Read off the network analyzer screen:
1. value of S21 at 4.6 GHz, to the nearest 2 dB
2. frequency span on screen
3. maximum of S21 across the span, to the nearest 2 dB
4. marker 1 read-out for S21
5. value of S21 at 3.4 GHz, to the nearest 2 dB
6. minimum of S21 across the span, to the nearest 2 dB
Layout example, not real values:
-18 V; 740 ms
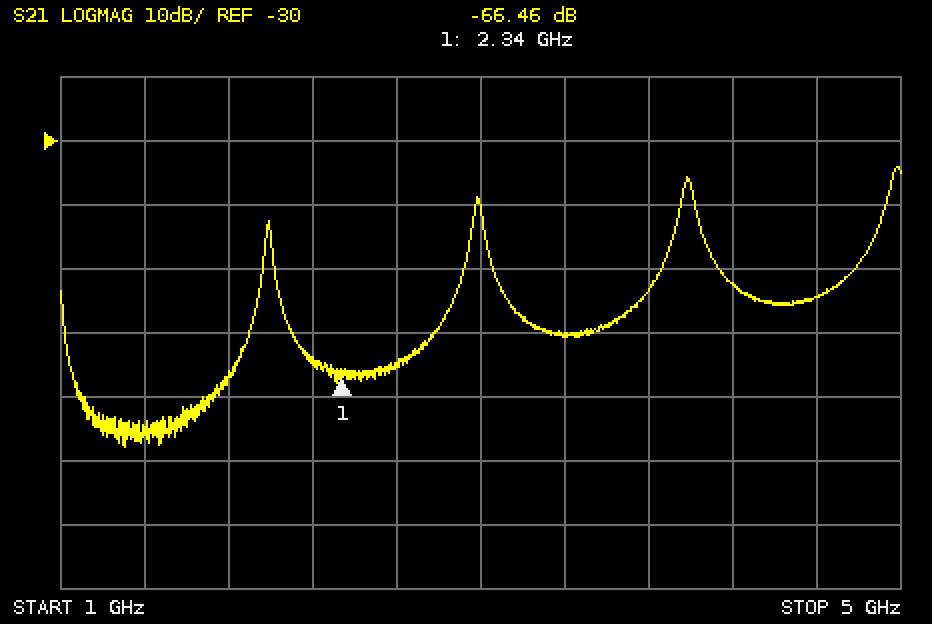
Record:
-54 dB; 4 GHz; -34 dB; -66.46 dB; -60 dB; -78 dB
